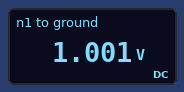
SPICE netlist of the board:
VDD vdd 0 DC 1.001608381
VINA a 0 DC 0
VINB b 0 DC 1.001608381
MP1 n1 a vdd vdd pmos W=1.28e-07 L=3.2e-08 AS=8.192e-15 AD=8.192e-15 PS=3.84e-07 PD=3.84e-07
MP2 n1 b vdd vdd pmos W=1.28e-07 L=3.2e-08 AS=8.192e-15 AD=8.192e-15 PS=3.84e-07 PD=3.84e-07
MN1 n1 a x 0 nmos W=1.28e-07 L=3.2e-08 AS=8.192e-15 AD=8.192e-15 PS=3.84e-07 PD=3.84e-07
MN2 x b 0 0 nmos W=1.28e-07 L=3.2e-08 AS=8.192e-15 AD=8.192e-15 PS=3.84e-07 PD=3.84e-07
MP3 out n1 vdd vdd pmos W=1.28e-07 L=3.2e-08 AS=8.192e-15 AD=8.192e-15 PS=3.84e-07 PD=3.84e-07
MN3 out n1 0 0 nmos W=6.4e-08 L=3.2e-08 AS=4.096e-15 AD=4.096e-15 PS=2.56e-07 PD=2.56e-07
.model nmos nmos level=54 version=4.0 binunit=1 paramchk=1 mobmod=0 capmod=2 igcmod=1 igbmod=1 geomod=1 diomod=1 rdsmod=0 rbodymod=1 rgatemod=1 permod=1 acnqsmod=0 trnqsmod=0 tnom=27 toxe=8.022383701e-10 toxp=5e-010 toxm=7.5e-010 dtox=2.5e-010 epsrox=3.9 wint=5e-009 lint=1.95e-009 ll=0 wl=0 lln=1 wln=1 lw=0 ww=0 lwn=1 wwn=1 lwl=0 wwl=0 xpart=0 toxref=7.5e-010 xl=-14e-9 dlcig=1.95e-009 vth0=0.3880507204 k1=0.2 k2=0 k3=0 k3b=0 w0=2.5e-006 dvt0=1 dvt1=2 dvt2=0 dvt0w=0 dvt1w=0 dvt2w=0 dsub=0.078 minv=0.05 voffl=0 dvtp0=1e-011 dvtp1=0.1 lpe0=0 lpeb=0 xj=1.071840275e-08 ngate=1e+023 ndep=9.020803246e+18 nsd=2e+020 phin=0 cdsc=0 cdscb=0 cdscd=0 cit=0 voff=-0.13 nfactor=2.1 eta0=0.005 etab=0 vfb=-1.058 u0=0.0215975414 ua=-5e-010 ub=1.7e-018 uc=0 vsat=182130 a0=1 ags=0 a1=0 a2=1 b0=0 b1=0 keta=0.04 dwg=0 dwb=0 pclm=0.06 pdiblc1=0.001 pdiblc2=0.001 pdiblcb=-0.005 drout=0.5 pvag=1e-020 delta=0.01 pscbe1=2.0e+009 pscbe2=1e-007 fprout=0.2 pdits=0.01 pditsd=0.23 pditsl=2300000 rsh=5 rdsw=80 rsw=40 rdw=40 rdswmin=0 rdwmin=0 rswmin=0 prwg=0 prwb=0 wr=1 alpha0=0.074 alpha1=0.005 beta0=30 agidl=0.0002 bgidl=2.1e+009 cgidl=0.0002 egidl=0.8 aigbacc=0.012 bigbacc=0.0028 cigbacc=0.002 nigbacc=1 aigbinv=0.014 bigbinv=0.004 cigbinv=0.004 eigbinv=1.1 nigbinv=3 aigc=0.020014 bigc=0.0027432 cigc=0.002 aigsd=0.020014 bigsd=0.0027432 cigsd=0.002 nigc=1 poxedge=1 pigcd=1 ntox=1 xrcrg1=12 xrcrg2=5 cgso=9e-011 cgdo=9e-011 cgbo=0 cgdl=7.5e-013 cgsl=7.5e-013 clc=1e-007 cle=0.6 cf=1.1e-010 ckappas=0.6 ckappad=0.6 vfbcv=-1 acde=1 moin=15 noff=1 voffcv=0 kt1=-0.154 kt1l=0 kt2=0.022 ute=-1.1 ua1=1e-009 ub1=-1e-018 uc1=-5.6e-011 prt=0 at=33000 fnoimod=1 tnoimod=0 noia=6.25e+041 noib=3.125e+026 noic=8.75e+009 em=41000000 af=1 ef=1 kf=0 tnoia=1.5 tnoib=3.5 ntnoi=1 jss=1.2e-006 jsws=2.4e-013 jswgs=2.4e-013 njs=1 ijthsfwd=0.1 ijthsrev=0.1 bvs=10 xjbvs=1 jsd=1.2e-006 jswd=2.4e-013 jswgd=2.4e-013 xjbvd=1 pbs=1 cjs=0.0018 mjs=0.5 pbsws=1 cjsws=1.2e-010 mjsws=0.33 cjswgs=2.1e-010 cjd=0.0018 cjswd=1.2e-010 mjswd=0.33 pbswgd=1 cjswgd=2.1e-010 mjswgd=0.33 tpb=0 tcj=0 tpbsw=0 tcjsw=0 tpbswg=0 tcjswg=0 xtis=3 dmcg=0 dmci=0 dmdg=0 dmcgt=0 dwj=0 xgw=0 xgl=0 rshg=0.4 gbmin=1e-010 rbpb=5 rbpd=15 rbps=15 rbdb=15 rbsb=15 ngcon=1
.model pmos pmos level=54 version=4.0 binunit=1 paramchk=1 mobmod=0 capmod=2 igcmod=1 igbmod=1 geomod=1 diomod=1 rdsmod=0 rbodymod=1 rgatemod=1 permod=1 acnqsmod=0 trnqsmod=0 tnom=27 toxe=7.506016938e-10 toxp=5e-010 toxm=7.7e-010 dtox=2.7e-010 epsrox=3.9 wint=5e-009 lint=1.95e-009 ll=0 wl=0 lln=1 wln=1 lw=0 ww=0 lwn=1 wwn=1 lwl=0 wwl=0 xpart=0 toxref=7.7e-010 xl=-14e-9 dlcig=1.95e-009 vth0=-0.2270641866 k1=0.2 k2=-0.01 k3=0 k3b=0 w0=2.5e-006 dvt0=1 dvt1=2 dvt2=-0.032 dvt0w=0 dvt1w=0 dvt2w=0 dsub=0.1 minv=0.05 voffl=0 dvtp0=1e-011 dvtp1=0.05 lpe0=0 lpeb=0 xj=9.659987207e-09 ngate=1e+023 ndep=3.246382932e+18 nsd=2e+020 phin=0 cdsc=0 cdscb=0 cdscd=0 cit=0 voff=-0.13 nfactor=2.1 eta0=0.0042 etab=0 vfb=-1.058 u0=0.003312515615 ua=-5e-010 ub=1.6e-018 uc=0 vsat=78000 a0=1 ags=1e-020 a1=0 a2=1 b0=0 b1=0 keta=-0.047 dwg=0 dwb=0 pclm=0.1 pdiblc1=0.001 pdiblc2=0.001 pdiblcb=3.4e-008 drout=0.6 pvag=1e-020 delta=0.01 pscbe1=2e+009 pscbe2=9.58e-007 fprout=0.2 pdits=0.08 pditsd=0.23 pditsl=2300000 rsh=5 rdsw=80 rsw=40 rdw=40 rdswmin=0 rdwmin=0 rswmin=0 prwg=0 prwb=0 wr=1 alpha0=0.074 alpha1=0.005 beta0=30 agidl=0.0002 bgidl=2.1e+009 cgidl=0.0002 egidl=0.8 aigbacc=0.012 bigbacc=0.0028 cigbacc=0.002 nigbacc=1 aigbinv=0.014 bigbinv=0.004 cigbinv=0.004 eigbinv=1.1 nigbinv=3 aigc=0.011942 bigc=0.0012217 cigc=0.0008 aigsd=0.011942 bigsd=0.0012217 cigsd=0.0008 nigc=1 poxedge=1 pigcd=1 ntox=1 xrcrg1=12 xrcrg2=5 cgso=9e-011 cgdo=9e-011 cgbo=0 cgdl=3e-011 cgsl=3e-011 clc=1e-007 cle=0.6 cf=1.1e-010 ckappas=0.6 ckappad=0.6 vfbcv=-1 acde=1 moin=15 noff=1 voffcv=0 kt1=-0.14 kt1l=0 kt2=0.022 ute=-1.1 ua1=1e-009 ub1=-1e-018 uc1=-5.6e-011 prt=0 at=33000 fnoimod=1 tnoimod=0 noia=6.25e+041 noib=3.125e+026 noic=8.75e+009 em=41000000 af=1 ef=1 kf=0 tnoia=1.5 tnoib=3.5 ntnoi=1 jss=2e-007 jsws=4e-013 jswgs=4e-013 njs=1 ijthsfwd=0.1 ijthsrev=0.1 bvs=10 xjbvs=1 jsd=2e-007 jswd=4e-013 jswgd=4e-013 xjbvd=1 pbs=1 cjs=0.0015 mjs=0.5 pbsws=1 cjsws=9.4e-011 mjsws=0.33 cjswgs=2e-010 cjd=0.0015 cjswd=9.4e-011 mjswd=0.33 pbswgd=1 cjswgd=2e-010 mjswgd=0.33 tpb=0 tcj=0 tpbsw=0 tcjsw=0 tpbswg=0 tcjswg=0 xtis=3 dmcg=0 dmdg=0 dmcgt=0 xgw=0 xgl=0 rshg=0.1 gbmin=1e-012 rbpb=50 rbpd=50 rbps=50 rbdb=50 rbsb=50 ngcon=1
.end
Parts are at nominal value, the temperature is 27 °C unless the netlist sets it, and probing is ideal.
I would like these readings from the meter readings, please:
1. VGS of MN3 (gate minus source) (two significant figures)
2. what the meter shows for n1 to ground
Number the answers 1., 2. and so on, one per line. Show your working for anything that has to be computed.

1. 1.001 V = 1.0 V
2. 1.001 V
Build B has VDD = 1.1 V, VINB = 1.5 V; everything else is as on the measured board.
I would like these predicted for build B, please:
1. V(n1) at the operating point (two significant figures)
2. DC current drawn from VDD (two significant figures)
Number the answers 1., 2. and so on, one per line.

1. 1.1 V
2. 350 nA
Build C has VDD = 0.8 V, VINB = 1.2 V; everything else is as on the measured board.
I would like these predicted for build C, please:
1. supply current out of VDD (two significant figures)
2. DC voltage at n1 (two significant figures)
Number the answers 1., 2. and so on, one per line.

1. 120 nA
2. 800 mV
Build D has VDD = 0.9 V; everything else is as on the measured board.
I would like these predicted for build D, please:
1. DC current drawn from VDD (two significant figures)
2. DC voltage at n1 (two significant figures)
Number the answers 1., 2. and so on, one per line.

1. 170 nA
2. 900 mV
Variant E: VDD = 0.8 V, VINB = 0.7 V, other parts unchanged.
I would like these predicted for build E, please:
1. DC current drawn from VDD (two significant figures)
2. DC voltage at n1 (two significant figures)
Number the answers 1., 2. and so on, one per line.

1. 120 nA
2. 800 mV
